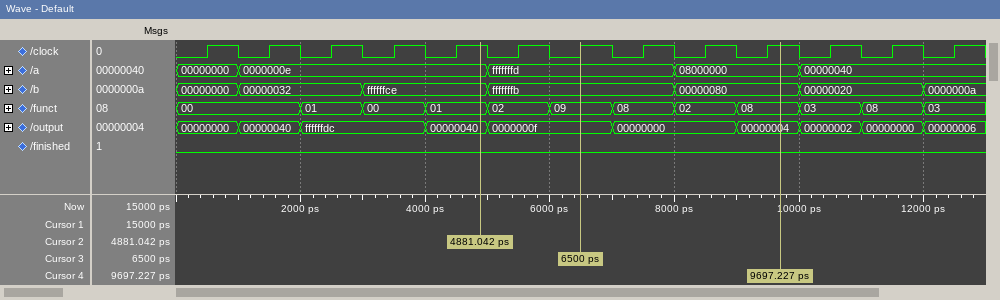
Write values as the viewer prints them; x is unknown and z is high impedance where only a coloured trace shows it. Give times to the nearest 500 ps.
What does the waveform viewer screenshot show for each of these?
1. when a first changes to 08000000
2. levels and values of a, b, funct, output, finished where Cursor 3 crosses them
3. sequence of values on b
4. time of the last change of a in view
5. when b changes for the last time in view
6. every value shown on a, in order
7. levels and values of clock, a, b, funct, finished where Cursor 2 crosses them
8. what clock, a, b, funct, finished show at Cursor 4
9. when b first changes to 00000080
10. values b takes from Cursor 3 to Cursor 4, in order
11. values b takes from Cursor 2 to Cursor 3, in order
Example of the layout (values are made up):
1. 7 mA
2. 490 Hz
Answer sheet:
1. 8000 ps
2. a=fffffffd, b=fffffffb, funct=09, output=0000000f, finished=0
3. 00000000, 00000032, ffffffce, fffffffb, 00000080, 00000020, 0000000a
4. 10000 ps
5. 12000 ps
6. 00000000, 0000000e, fffffffd, 08000000, 00000040
7. clock=1, a=0000000e, b=ffffffce, funct=01, finished=0
8. clock=1, a=08000000, b=00000080, funct=08, finished=0
9. 8000 ps
10. fffffffb, 00000080
11. ffffffce, fffffffb
